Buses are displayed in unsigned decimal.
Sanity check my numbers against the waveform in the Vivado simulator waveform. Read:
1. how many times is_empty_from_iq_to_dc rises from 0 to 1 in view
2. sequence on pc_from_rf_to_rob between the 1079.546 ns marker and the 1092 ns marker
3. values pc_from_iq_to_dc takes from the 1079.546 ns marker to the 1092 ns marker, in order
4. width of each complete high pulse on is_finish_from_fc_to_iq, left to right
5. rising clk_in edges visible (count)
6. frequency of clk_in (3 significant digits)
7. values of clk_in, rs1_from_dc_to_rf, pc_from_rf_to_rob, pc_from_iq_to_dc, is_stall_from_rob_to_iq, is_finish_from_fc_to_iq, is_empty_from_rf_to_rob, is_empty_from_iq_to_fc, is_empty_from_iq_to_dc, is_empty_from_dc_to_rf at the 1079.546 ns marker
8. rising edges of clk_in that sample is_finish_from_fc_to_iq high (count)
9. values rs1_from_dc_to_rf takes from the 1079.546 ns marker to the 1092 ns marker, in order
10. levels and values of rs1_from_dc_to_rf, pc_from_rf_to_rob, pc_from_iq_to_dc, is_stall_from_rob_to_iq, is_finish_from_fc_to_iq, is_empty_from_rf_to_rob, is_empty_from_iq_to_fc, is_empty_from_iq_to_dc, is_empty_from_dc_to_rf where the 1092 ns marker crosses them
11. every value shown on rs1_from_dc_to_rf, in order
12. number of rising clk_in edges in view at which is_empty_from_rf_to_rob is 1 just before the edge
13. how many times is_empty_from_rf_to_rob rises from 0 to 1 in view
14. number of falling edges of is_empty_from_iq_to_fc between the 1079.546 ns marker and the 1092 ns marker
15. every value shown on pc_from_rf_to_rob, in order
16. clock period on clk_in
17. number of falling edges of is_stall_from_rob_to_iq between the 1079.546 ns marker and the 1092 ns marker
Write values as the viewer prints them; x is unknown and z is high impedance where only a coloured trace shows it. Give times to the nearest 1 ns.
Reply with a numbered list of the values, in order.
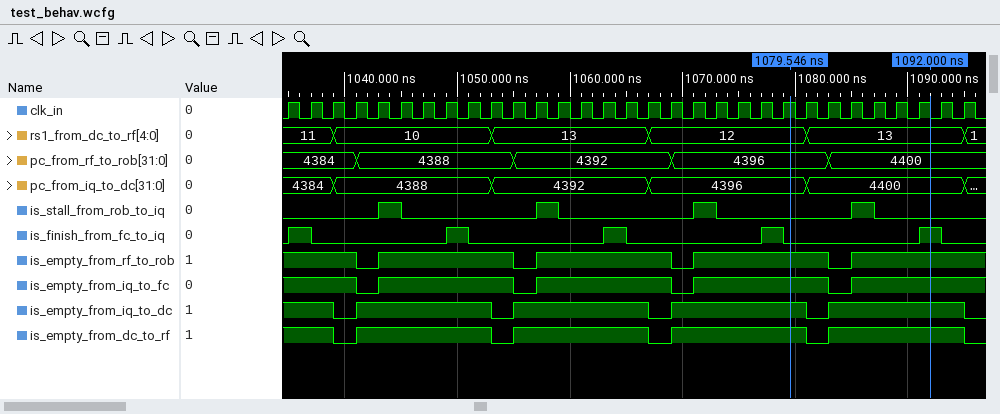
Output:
1. 4
2. 4396, 4400
3. 4396, 4400
4. 2 ns, 2 ns, 2 ns, 2 ns, 2 ns
5. 31
6. 500 MHz
7. clk_in=1, rs1_from_dc_to_rf=12, pc_from_rf_to_rob=4396, pc_from_iq_to_dc=4396, is_stall_from_rob_to_iq=0, is_finish_from_fc_to_iq=0, is_empty_from_rf_to_rob=1, is_empty_from_iq_to_fc=1, is_empty_from_iq_to_dc=1, is_empty_from_dc_to_rf=1
8. 5
9. 12, 13
10. rs1_from_dc_to_rf=13, pc_from_rf_to_rob=4400, pc_from_iq_to_dc=4400, is_stall_from_rob_to_iq=0, is_finish_from_fc_to_iq=1, is_empty_from_rf_to_rob=1, is_empty_from_iq_to_fc=1, is_empty_from_iq_to_dc=1, is_empty_from_dc_to_rf=1
11. 11, 10, 13, 12, 13, 1
12. 27
13. 4
14. 1
15. 4384, 4388, 4392, 4396, 4400
16. 2 ns
17. 1
